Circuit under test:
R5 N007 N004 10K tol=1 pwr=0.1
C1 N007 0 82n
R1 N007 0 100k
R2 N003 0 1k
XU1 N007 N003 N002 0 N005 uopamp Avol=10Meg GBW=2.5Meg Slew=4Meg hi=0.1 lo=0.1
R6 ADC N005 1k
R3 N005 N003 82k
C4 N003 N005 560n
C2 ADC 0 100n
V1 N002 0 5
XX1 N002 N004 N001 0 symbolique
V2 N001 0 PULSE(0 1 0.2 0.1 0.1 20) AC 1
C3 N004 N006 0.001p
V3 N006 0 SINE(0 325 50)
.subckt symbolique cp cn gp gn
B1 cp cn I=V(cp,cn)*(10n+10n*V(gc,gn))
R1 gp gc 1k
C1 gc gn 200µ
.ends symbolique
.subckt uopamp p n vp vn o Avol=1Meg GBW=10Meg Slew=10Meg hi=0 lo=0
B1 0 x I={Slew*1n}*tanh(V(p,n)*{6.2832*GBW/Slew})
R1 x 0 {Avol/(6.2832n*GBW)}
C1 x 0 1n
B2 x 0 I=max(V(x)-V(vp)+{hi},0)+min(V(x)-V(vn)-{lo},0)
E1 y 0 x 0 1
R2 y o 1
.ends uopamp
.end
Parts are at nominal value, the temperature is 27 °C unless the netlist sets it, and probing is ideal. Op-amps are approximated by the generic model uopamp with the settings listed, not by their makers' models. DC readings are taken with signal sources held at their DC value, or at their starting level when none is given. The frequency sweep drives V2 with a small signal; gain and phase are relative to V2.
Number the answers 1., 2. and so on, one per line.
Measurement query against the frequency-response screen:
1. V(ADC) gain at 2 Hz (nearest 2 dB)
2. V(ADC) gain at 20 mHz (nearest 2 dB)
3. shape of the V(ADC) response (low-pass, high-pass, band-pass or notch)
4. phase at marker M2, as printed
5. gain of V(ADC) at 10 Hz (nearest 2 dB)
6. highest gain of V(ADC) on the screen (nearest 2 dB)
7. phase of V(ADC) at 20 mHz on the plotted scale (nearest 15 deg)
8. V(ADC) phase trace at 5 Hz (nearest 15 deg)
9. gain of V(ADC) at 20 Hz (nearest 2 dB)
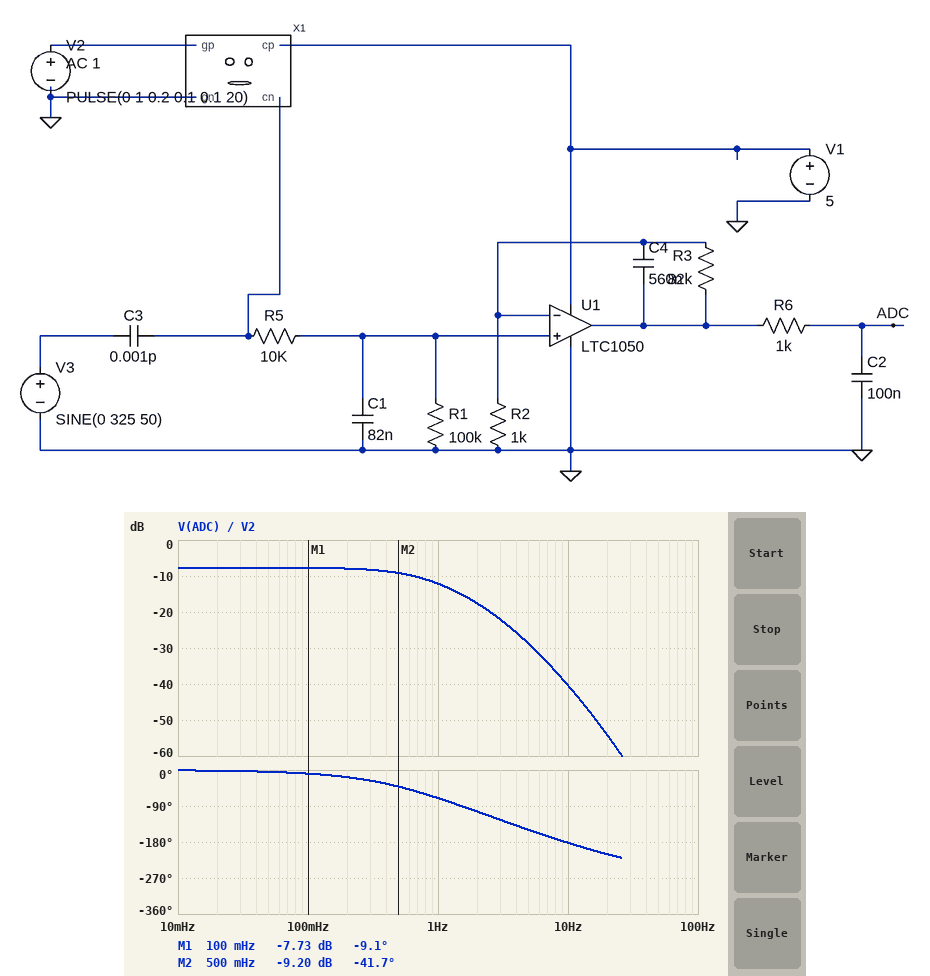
1. -18 dB
2. -8 dB
3. low-pass
4. -41.7 deg
5. -40 dB
6. -8 dB
7. 0 deg
8. -150 deg
9. -54 dB
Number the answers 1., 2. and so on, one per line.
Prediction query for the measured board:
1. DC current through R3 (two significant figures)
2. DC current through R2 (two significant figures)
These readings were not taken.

1. 5.0 µA
2. 5.0 µA
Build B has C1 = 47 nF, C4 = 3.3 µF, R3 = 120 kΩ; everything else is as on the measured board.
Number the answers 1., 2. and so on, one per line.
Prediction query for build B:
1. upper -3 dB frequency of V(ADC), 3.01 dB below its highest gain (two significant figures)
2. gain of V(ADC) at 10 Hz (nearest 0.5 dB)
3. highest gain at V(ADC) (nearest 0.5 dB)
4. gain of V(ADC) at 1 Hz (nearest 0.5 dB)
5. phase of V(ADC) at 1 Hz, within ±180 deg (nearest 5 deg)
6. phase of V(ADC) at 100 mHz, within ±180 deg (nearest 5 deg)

1. 340 mHz
2. -54.5 dB
3. -4.5 dB
4. -17.0 dB
5. -120 deg
6. -20 deg
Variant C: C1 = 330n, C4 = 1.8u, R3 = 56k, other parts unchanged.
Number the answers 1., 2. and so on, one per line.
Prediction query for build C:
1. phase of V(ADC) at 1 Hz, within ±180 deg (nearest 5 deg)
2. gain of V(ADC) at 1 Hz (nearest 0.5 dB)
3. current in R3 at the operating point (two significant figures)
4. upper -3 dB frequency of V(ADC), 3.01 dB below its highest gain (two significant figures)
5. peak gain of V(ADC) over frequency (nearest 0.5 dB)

1. -95 deg
2. -16.5 dB
3. 5.0 µA
4. 650 mHz
5. -11.0 dB
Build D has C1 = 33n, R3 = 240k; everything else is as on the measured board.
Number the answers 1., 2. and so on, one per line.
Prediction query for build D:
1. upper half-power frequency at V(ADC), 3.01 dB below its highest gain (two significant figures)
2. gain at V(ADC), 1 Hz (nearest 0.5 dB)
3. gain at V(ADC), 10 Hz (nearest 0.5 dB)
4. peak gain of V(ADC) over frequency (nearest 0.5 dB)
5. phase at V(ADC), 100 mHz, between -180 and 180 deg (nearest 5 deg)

1. 610 mHz
2. -5.0 dB
3. -39.0 dB
4. 1.5 dB
5. -10 deg
